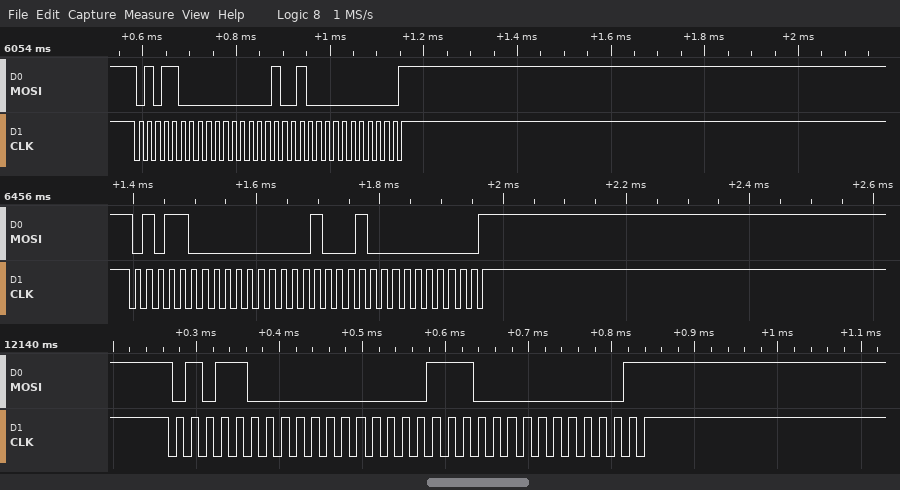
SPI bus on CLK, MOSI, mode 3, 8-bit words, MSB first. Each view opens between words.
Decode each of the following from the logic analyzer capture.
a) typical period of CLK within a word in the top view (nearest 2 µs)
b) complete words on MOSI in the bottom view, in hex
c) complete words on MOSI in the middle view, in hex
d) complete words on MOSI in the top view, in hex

18 µs
58, 00, 70, 03
58, 00, 88, 01
58, 00, 90, 01
